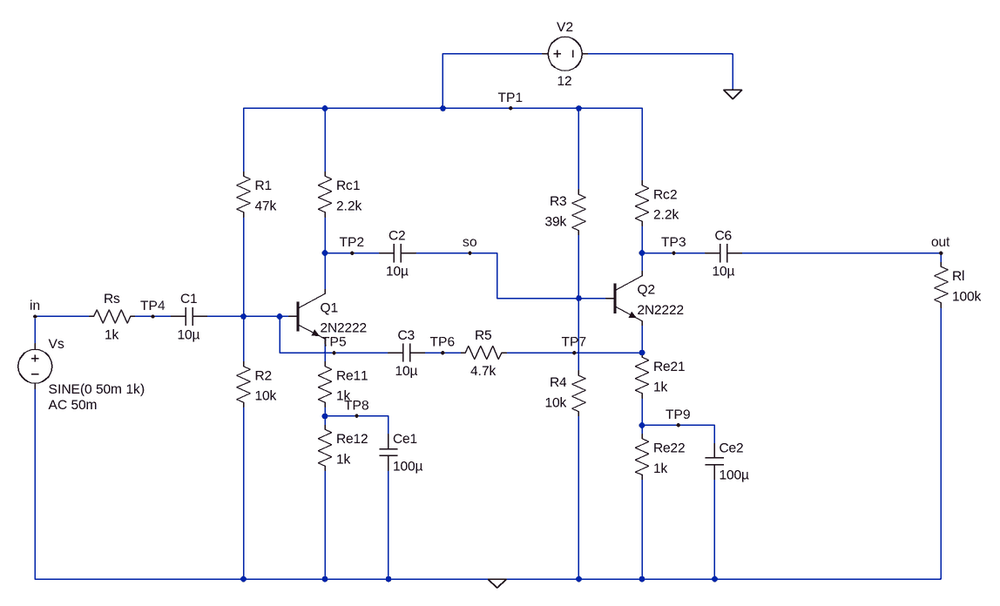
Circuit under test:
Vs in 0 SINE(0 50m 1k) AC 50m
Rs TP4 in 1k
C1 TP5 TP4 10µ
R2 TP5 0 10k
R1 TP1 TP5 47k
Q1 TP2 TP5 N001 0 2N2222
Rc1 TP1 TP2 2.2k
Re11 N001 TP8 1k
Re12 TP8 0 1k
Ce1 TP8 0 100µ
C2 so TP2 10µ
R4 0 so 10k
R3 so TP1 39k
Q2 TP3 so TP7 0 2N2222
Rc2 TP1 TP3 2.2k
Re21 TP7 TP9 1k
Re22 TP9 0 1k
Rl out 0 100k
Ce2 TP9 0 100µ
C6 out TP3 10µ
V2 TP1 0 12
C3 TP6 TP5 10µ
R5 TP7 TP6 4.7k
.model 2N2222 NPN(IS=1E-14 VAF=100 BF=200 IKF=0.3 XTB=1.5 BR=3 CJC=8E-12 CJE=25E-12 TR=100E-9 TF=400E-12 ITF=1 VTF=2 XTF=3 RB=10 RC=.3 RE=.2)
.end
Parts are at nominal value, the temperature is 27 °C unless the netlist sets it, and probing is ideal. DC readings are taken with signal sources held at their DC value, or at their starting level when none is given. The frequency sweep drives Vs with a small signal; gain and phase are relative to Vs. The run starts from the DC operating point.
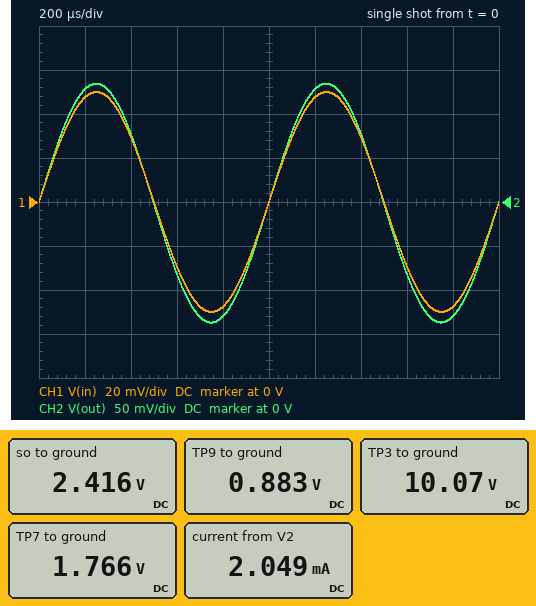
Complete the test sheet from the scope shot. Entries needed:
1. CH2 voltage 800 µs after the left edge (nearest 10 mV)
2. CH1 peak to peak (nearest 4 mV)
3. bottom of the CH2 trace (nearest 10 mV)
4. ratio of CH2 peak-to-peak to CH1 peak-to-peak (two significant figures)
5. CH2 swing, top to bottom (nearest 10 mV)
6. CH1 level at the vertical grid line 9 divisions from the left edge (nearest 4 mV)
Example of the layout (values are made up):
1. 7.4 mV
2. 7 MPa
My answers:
1. -130 mV
2. 100 mV
3. -140 mV
4. 2.7
5. 270 mV
6. -48 mV
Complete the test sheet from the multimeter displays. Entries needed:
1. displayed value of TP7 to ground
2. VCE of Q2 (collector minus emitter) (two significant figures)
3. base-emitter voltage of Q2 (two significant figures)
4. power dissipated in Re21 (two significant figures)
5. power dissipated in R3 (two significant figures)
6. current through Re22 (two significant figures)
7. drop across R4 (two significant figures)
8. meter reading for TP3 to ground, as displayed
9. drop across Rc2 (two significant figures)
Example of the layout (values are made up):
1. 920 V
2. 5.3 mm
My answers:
1. 1.766 V
2. 8.3 V
3. 650 mV
4. 780 µW
5. 2.4 mW
6. 880 µA
7. 2.4 V
8. 10.07 V
9. 1.9 V
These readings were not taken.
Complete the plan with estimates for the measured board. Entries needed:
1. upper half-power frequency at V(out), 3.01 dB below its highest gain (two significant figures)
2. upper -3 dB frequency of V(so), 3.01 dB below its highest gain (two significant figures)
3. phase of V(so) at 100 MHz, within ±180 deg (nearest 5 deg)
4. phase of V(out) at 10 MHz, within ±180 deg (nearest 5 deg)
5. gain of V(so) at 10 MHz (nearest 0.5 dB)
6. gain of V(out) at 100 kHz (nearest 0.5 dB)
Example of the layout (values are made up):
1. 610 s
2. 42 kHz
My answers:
1. 4.8 MHz
2. 5.1 MHz
3. 25 deg
4. -110 deg
5. -6.5 dB
6. 8.5 dB
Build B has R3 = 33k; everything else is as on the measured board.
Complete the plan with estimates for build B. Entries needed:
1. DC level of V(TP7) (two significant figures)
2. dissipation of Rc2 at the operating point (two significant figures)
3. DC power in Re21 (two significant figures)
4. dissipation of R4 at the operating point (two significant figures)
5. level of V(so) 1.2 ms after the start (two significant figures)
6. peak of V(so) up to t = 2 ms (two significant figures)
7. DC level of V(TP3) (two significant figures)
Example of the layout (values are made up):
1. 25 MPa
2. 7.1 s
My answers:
1. 2.1 V
2. 2.4 mW
3. 1.1 mW
4. 760 µW
5. 2.7 V
6. 2.8 V
7. 9.7 V
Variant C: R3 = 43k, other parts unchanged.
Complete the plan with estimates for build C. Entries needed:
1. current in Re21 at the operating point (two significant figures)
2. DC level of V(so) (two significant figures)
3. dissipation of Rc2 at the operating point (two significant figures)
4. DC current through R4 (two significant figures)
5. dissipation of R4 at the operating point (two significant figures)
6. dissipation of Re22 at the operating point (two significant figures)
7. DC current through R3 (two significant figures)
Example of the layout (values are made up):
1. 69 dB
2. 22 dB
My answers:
1. 790 µA
2. 2.2 V
3. 1.4 mW
4. 220 µA
5. 500 µW
6. 630 µW
7. 230 µA
